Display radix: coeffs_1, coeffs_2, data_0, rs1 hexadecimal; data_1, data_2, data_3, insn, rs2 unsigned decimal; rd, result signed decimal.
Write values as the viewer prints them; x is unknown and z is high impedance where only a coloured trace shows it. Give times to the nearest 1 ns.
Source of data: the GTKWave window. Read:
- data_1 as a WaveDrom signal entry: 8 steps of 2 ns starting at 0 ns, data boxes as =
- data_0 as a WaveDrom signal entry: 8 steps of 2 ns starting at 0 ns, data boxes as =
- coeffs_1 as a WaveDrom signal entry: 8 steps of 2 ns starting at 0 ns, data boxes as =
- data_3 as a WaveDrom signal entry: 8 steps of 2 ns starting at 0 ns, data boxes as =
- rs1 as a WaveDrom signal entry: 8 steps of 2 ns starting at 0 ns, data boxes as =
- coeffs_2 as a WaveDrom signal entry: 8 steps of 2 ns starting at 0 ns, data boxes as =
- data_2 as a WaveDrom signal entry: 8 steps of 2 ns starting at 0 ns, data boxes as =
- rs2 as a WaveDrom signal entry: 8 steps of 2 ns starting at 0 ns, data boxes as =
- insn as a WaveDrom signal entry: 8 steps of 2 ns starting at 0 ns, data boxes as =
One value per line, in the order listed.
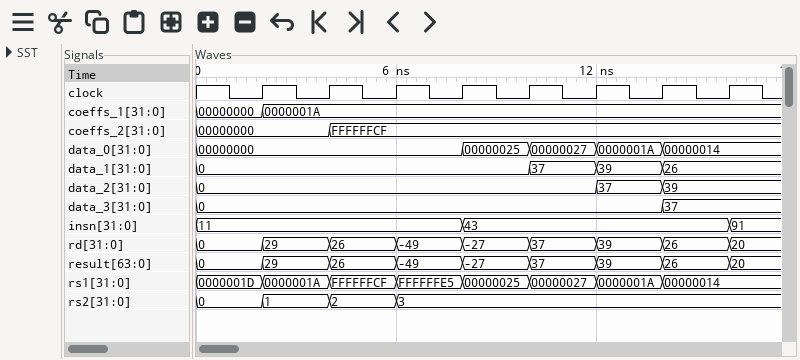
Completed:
{name: 'data_1', wave: '=....===', data: '0 37 39 26'}
{name: 'data_0', wave: '=...====', data: '00000000 00000025 00000027 0000001A 00000014'}
{name: 'coeffs_1', wave: '==......', data: '00000000 0000001A'}
{name: 'data_3', wave: '=......=', data: '0 37'}
{name: 'rs1', wave: '========', data: '0000001D 0000001A FFFFFFCF FFFFFFE5 00000025 00000027 0000001A 00000014'}
{name: 'coeffs_2', wave: '=.=.....', data: '00000000 FFFFFFCF'}
{name: 'data_2', wave: '=.....==', data: '0 37 39'}
{name: 'rs2', wave: '====....', data: '0 1 2 3'}
{name: 'insn', wave: '=...=...', data: '11 43'}
